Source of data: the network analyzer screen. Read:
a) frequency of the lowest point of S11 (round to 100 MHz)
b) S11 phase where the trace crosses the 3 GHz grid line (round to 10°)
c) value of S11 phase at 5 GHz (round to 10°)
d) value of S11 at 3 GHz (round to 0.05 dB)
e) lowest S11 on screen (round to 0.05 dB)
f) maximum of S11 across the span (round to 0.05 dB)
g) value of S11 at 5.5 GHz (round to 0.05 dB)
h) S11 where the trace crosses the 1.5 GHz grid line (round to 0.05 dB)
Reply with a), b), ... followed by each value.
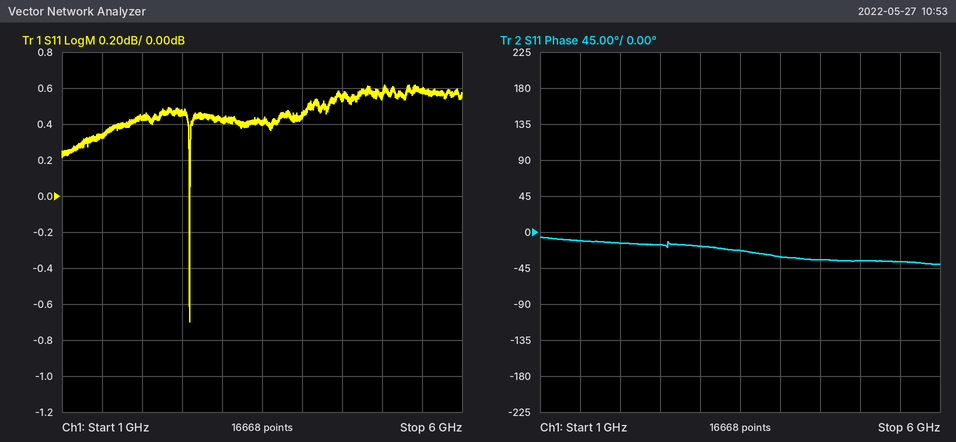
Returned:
a) 2.6 GHz
b) -20°
c) -40°
d) 0.40 dB
e) -0.70 dB
f) 0.60 dB
g) 0.60 dB
h) 0.35 dB
